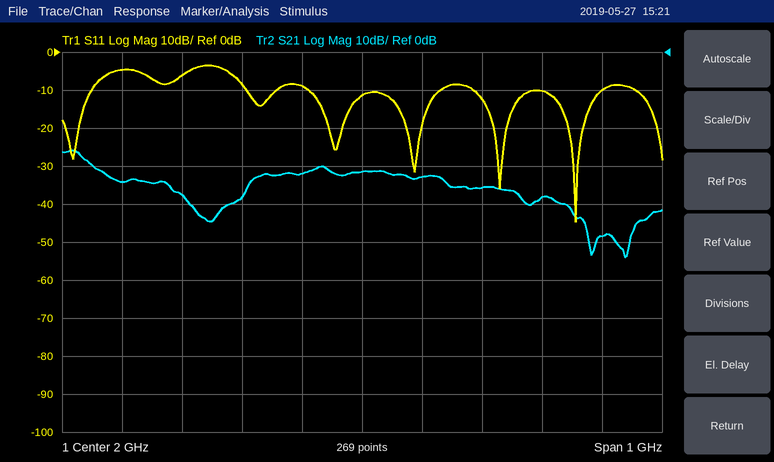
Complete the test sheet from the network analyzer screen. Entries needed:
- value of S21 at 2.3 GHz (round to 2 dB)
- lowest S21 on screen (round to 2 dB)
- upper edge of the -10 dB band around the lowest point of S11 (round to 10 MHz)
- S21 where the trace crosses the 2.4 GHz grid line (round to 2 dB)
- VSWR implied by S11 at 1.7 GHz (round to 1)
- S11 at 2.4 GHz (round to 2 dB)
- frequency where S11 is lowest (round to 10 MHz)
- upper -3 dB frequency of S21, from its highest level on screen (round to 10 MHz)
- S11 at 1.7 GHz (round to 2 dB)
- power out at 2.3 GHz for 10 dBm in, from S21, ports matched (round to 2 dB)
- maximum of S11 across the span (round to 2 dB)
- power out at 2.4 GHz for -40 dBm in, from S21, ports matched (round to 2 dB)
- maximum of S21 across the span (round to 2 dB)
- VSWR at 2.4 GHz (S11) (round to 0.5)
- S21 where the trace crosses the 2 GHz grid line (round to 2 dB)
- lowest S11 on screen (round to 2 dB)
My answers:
-38 dB
-54 dB
2.40 GHz
-48 dB
3
-10 dB
2.36 GHz
1.54 GHz
-6 dB
-28 dBm
-4 dB
-88 dBm
-26 dB
2.0
-32 dB
-44 dB
